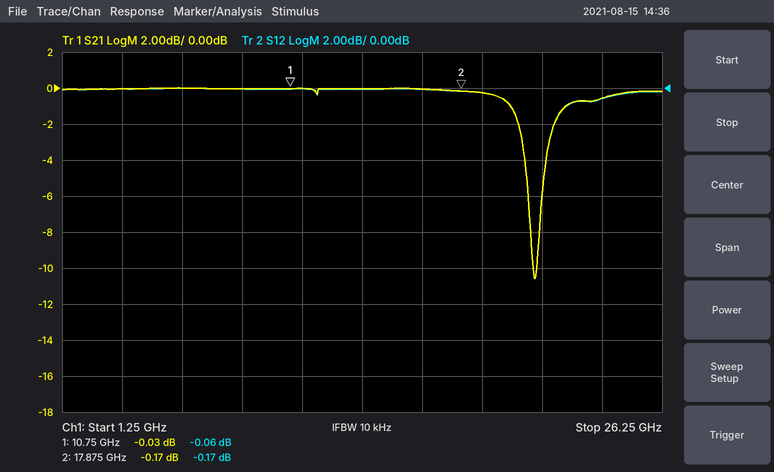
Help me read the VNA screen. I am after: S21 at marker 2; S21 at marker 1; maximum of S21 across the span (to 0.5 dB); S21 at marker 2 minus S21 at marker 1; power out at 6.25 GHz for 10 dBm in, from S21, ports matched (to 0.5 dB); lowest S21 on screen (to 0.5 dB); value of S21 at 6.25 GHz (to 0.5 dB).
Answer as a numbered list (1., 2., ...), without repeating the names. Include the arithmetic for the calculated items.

1. -0.17 dB
2. -0.03 dB
3. 0.0 dB
4. -0.17 − (-0.03) = -0.14 dB
5. 10 dBm + (0.0 dB) = 10.0 dBm
6. -10.5 dB
7. 0.0 dB
